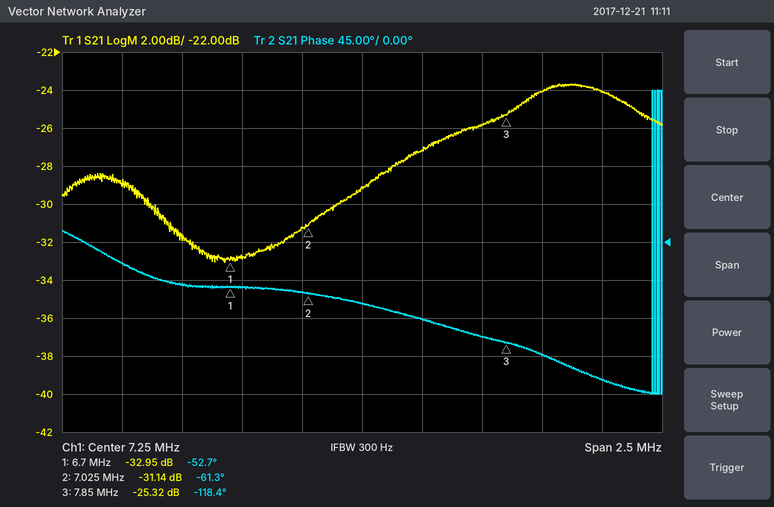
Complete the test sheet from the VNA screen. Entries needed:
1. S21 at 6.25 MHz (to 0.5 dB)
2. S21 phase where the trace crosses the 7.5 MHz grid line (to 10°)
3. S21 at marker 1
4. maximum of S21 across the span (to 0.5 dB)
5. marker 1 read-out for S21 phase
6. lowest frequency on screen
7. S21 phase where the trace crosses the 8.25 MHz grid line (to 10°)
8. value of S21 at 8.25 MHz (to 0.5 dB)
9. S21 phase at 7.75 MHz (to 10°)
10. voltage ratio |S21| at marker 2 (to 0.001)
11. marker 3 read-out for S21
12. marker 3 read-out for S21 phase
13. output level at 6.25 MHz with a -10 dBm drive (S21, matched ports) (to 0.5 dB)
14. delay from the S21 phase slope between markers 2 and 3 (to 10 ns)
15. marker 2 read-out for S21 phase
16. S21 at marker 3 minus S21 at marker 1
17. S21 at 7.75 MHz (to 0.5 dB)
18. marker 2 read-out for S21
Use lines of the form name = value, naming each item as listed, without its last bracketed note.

S21 at 6.25 MHz = -29.0 dB
S21 phase where the trace crosses the 7.5 MHz grid line = -90°
S21 at marker 1 = -32.95 dB
maximum of S21 across the span = -23.5 dB
marker 1 read-out for S21 phase = -52.7°
lowest frequency on screen = 6 MHz
S21 phase where the trace crosses the 8.25 MHz grid line = -160°
value of S21 at 8.25 MHz = -24.0 dB
S21 phase at 7.75 MHz = -110°
voltage ratio |S21| at marker 2 = 0.028
marker 3 read-out for S21 = -25.32 dB
marker 3 read-out for S21 phase = -118.4°
output level at 6.25 MHz with a -10 dBm drive (S21, matched ports) = -39.0 dBm
delay from the S21 phase slope between markers 2 and 3 = 190 ns
marker 2 read-out for S21 phase = -61.3°
S21 at marker 3 minus S21 at marker 1 = 7.63 dB
S21 at 7.75 MHz = -26.0 dB
marker 2 read-out for S21 = -31.14 dB
